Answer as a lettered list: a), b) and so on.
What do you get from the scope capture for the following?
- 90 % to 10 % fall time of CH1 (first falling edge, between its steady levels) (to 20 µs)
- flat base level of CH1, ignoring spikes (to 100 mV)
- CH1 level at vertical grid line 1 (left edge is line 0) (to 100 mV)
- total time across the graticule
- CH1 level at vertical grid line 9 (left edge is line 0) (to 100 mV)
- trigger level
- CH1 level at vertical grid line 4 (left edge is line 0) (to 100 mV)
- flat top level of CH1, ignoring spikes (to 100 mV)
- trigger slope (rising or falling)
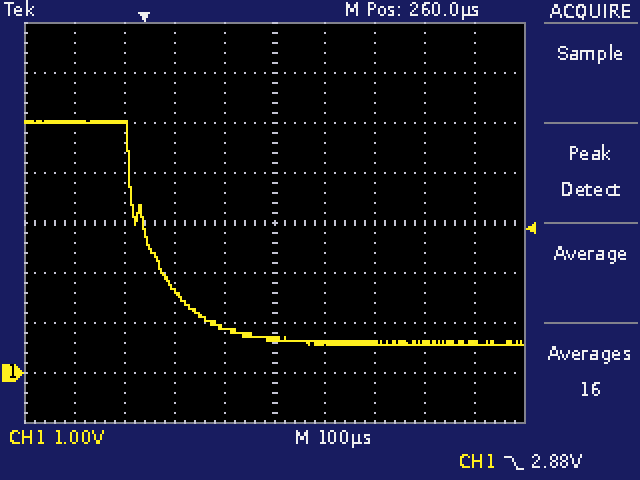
a) 160 µs
b) 600 mV
c) 5.0 V
d) 1 ms
e) 600 mV
f) 2.88 V
g) 900 mV
h) 5.0 V
i) falling
